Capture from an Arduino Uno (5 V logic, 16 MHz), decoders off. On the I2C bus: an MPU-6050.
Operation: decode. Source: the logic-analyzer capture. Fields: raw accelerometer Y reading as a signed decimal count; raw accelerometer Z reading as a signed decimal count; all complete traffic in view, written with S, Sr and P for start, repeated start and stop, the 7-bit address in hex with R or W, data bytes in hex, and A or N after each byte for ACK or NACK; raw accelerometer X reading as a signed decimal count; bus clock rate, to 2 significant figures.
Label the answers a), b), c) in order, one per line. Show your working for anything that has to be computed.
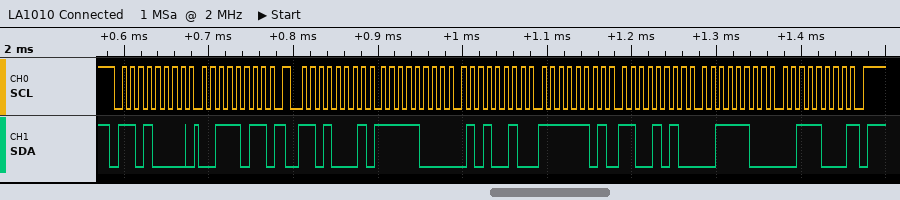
a) 0xFDCA = -566
b) 0x3C38 = 15416
c) S 68W A 3B A Sr 68R A F8 A 52 A FD A CA A 3C A 38 N P
d) 0xF852 = -1966
e) 100 kHz
